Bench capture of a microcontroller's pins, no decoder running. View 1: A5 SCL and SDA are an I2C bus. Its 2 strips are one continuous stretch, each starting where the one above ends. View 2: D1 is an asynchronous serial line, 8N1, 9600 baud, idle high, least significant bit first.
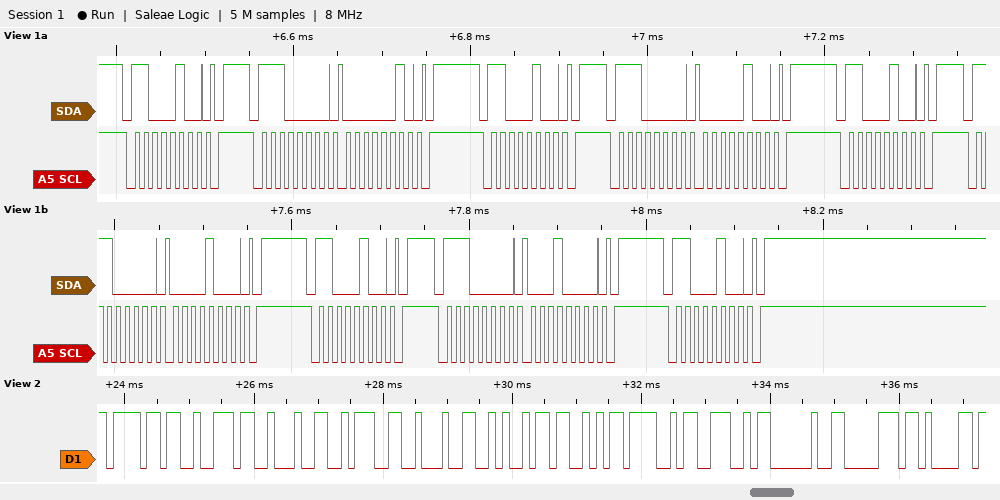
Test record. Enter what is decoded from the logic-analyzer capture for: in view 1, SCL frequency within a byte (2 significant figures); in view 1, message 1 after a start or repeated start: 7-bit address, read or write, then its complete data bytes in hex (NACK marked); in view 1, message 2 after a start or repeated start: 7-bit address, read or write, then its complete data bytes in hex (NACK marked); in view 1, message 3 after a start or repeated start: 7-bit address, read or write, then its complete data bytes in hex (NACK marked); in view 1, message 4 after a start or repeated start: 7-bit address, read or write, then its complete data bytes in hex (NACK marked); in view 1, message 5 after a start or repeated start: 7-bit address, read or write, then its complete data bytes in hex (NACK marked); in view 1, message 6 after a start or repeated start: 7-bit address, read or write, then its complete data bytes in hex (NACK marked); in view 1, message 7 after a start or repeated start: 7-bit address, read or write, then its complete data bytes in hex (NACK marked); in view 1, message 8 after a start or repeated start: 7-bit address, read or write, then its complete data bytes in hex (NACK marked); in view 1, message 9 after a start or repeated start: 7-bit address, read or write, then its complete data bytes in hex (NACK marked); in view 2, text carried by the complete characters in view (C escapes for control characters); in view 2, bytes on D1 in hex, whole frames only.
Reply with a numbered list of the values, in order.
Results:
1. 100 kHz
2. 0x62 write
3. 0x70 write: 02
4. 0x62 write
5. 0x70 write: 04
6. 0x62 write
7. 0x70 write: 08
8. 0x62 write
9. 0x70 write: 10
10. 0x62 write
11. "or\":\"JSON pa"
12. 6F 72 22 3A 22 4A 53 4F 4E 20 70 61
